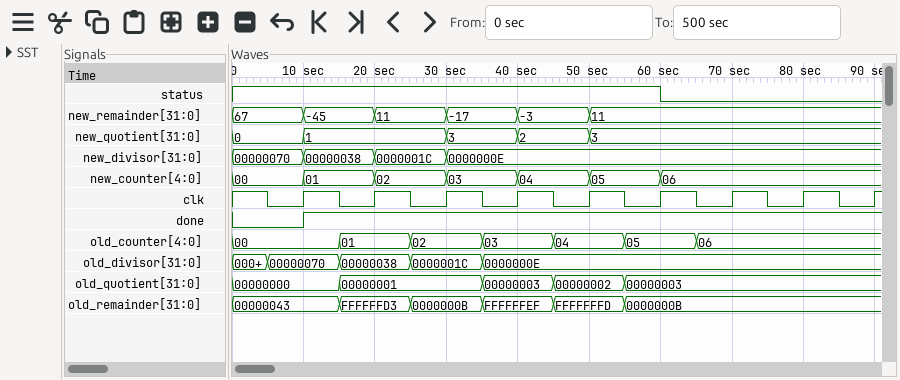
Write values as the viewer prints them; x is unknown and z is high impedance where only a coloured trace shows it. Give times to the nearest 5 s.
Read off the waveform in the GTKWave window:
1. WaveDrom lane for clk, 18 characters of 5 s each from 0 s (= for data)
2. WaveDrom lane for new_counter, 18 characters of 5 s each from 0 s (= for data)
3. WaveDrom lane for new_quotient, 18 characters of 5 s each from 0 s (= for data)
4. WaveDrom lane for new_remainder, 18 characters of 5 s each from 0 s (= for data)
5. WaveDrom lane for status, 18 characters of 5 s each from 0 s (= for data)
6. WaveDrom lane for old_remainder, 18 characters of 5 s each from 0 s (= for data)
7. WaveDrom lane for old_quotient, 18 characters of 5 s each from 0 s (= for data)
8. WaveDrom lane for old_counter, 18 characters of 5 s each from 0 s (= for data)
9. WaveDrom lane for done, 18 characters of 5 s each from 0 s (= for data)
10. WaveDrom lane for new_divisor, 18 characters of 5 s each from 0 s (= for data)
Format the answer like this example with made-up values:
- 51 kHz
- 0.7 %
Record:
- {name: 'clk', wave: '101010101010101010'}
- {name: 'new_counter', wave: '=.=.=.=.=.=.=.....', data: '00 01 02 03 04 05 06'}
- {name: 'new_quotient', wave: '=.=...=.=.=.......', data: '0 1 3 2 3'}
- {name: 'new_remainder', wave: '=.=.=.=.=.=.......', data: '67 -45 11 -17 -3 11'}
- {name: 'status', wave: '1...........0.....'}
- {name: 'old_remainder', wave: '=..=.=.=.=.=......', data: '00000043 FFFFFFD3 0000000B FFFFFFEF FFFFFFFD 0000000B'}
- {name: 'old_quotient', wave: '=..=...=.=.=......', data: '00000000 00000001 00000003 00000002 00000003'}
- {name: 'old_counter', wave: '=..=.=.=.=.=.=....', data: '00 01 02 03 04 05 06'}
- {name: 'done', wave: '0.1...............'}
- {name: 'new_divisor', wave: '=.=.=.=...........', data: '00000070 00000038 0000001C 0000000E'}
